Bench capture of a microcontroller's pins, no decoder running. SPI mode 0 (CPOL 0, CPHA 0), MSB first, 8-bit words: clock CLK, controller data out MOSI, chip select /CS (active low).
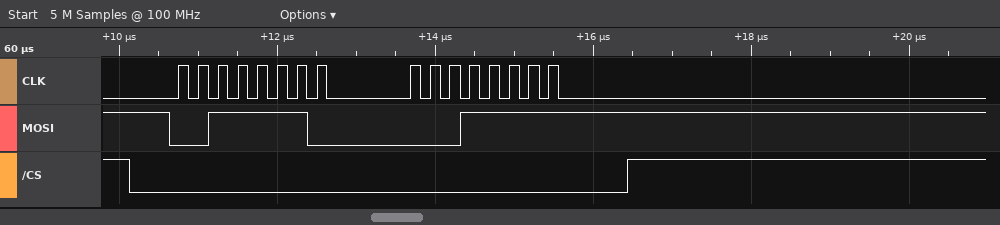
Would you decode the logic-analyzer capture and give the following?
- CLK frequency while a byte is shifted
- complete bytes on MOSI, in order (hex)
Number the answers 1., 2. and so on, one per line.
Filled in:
1. 4 MHz
2. 3E 1F
